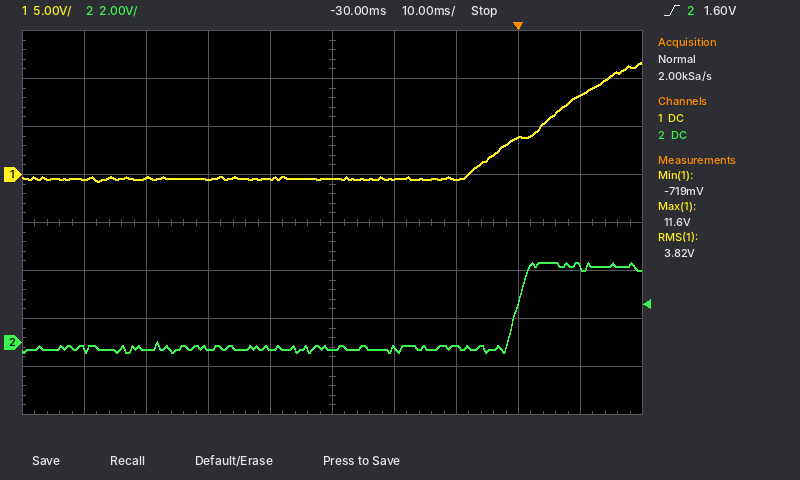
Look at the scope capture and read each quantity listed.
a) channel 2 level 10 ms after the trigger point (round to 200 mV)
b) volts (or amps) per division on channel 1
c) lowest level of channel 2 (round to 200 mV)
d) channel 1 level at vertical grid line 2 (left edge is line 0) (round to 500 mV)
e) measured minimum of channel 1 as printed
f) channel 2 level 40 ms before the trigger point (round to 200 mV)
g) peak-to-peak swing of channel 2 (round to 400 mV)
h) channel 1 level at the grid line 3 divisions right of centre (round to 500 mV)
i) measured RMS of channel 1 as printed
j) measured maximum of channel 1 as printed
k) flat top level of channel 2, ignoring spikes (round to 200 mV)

3.2 V
5 V
-400 mV
-500 mV
-719 mV
-200 mV
3.6 V
4.0 V
3.82 V
11.6 V
3.2 V
